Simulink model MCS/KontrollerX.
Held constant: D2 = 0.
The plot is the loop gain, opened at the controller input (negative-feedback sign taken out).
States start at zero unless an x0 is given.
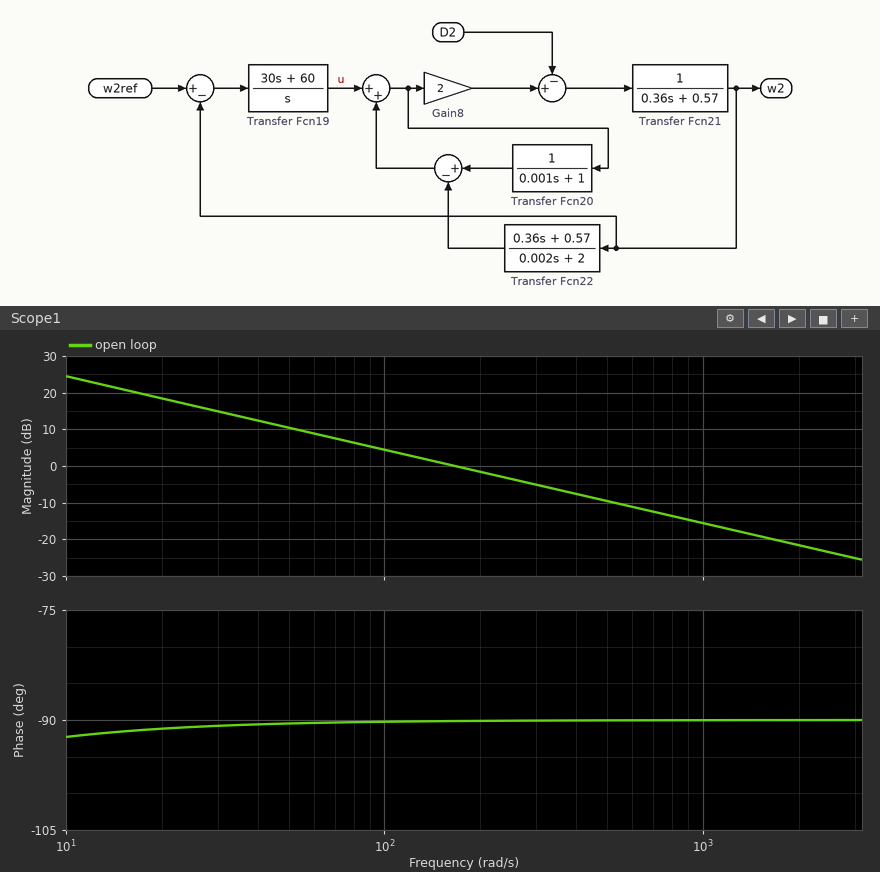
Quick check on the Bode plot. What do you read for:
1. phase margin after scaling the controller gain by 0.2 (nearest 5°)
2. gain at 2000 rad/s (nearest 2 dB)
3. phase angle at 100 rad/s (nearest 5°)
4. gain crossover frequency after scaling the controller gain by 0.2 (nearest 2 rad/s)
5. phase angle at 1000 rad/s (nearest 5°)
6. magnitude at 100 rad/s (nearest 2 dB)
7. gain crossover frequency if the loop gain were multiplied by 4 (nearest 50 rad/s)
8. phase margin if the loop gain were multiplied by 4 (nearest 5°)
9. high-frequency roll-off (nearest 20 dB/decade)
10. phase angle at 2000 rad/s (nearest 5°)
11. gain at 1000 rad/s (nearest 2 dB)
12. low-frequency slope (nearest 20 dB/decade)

90°
-22 dB
-90°
34 rad/s
-90°
4 dB
650 rad/s
90°
-20 dB/decade
-90°
-16 dB
-20 dB/decade
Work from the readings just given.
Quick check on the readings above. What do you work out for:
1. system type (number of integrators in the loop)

1
